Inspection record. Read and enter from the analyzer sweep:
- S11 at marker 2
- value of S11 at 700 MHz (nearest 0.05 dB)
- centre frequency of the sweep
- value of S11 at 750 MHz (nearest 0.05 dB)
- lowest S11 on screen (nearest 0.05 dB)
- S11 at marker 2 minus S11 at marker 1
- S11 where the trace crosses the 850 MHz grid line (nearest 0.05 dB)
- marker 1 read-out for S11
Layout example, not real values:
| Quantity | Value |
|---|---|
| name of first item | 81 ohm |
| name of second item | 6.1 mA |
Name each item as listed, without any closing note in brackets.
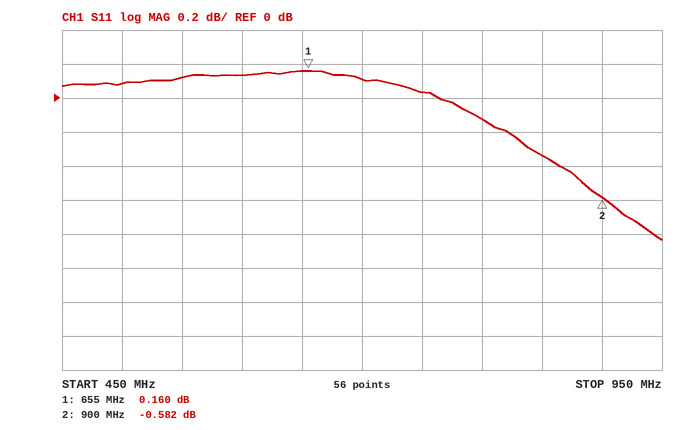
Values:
| Quantity | Value |
|---|---|
| S11 at marker 2 | -0.582 dB |
| value of S11 at 700 MHz | 0.10 dB |
| centre frequency of the sweep | 700 MHz |
| value of S11 at 750 MHz | 0.05 dB |
| lowest S11 on screen | -0.85 dB |
| S11 at marker 2 minus S11 at marker 1 | -0.742 dB |
| S11 where the trace crosses the 850 MHz grid line | -0.35 dB |
| marker 1 read-out for S11 | 0.160 dB |
